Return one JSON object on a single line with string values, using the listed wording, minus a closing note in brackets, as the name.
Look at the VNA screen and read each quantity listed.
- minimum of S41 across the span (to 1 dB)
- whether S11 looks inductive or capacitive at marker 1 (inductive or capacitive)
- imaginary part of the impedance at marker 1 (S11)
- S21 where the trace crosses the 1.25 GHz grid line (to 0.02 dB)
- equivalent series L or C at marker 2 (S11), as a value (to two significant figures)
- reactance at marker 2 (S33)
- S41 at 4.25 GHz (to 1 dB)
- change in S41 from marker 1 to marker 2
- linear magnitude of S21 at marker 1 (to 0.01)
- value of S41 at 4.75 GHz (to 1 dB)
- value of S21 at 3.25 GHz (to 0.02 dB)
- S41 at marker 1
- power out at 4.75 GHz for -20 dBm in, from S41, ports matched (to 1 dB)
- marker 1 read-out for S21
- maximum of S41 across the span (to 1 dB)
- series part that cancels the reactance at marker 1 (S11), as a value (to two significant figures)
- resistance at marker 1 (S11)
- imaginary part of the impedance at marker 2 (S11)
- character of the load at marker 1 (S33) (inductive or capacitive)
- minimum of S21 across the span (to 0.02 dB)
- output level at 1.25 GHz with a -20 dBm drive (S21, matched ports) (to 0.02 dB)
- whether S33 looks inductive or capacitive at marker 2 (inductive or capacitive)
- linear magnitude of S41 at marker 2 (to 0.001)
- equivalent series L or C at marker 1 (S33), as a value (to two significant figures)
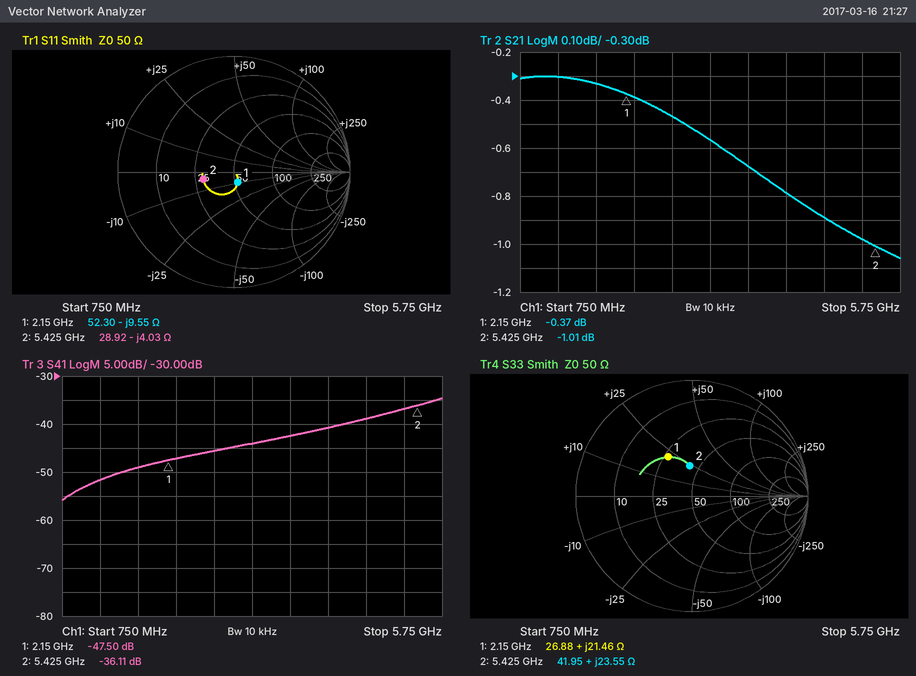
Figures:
{"minimum of S41 across the span": "-56 dB", "whether S11 looks inductive or capacitive at marker 1": "capacitive", "imaginary part of the impedance at marker 1": "-9.55 Ω", "S21 where the trace crosses the 1.25 GHz grid line": "-0.30 dB", "equivalent series L or C at marker 2 (S11), as a value": "7.3 pF", "reactance at marker 2": "+23.55 Ω", "S41 at 4.25 GHz": "-41 dB", "change in S41 from marker 1 to marker 2": "11.39 dB", "linear magnitude of S21 at marker 1": "0.96", "value of S41 at 4.75 GHz": "-39 dB", "value of S21 at 3.25 GHz": "-0.56 dB", "S41 at marker 1": "-47.50 dB", "power out at 4.75 GHz for -20 dBm in, from S41, ports matched": "-59 dBm", "marker 1 read-out for S21": "-0.37 dB", "maximum of S41 across the span": "-35 dB", "series part that cancels the reactance at marker 1 (S11), as a value": "710 pH", "resistance at marker 1": "52.30 Ω", "imaginary part of the impedance at marker 2": "-4.03 Ω", "character of the load at marker 1 (S33)": "inductive", "minimum of S21 across the span": "-1.06 dB", "output level at 1.25 GHz with a -20 dBm drive (S21, matched ports)": "-20.30 dBm", "whether S33 looks inductive or capacitive at marker 2": "inductive", "linear magnitude of S41 at marker 2": "0.016", "equivalent series L or C at marker 1 (S33), as a value": "1.6 nH"}
